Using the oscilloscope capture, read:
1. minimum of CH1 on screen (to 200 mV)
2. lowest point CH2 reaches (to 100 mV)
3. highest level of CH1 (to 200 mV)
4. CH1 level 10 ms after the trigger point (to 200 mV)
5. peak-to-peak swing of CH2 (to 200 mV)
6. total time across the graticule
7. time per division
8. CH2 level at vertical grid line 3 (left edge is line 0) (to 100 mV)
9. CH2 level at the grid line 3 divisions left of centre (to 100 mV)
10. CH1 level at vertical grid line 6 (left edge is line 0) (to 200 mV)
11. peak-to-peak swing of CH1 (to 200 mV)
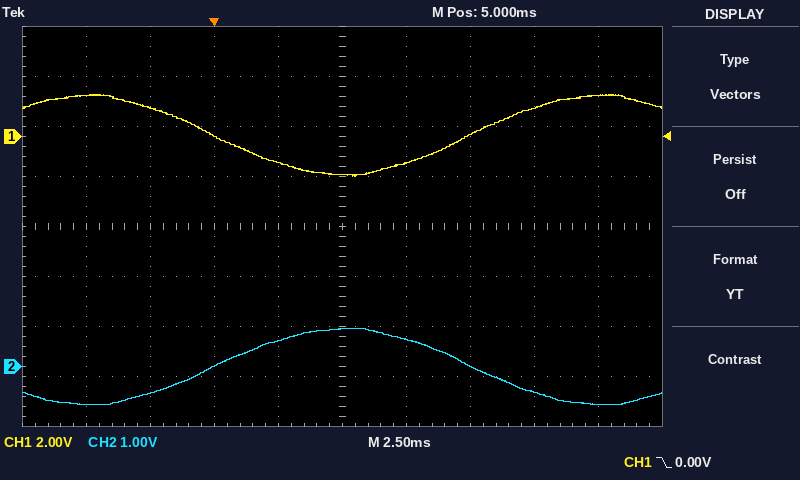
-1.6 V
-800 mV
1.6 V
0.0 V
1.6 V
25 ms
2.5 ms
0.0 V
-500 mV
-1.0 V
3.2 V
